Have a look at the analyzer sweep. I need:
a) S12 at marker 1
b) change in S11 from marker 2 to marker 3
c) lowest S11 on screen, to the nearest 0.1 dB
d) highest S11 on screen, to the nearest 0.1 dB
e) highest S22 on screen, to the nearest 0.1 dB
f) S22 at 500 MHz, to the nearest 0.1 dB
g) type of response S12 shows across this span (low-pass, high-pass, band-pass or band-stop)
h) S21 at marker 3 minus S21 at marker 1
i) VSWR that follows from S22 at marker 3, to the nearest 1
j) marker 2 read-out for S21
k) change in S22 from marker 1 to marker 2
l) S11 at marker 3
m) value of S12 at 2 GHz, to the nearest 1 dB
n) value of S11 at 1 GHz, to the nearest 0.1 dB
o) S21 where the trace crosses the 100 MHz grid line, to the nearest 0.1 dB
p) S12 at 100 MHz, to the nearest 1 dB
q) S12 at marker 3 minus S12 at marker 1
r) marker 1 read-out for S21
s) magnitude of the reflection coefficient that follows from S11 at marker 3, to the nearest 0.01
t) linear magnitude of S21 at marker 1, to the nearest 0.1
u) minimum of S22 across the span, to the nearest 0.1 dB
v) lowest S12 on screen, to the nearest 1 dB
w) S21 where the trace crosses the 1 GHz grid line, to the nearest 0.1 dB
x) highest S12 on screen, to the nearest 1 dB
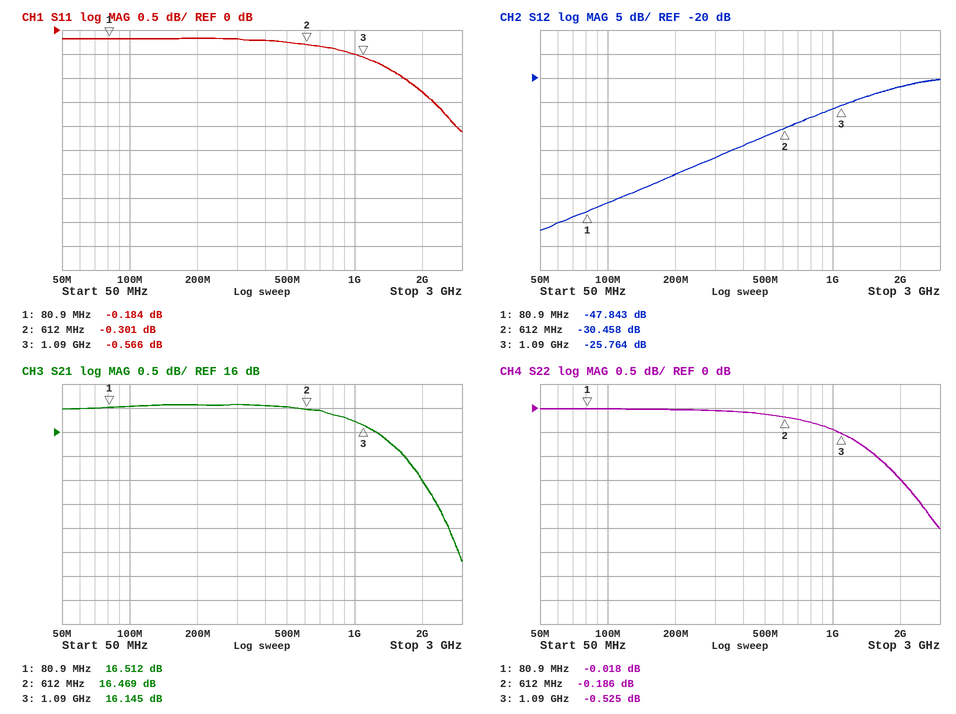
-47.843 dB
-0.265 dB
-2.1 dB
-0.2 dB
0.0 dB
-0.1 dB
high-pass
-0.367 dB
33
16.469 dB
-0.168 dB
-0.566 dB
-22 dB
-0.5 dB
16.5 dB
-46 dB
22.079 dB
16.512 dB
0.94
6.7
-2.5 dB
-52 dB
16.2 dB
-20 dB
